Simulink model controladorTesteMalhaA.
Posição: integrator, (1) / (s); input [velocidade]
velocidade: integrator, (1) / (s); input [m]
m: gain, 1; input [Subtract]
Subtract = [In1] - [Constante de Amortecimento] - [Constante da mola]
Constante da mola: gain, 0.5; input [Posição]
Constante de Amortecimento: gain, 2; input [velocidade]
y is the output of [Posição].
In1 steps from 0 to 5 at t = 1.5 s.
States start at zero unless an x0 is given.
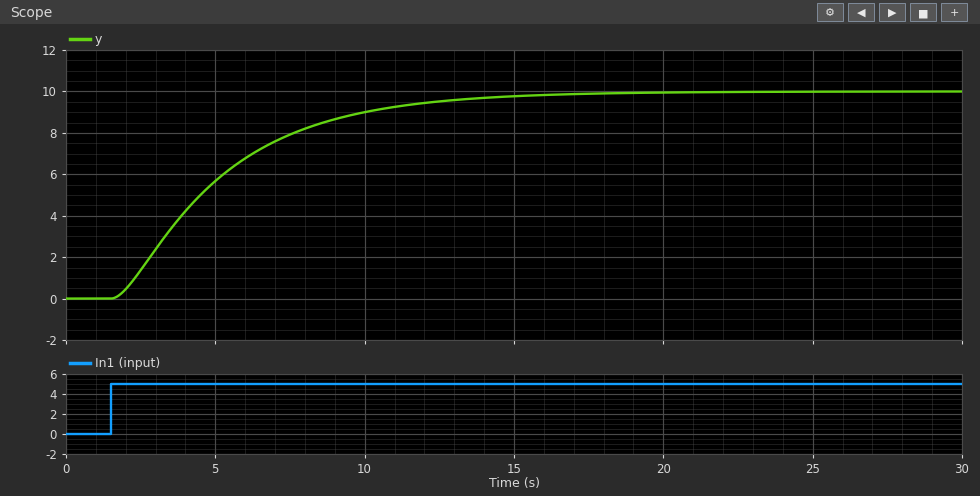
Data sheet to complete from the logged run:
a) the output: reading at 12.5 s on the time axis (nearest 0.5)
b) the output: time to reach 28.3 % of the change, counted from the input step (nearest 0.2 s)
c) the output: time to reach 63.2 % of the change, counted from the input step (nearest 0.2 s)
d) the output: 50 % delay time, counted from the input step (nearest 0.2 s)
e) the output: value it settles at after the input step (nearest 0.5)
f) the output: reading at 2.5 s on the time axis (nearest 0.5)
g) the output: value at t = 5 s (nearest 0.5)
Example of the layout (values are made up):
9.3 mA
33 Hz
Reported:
9.5
1.8 s
4.0 s
3.0 s
10.0
1.5
5.5
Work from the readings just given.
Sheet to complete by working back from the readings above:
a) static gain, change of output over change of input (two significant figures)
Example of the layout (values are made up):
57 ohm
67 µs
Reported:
2.0
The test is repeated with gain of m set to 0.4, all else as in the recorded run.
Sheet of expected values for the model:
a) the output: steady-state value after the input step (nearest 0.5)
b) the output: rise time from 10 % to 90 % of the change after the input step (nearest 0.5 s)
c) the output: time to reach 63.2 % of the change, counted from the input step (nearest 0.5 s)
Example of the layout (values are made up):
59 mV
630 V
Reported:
10.0
6.5 s
4.5 s
